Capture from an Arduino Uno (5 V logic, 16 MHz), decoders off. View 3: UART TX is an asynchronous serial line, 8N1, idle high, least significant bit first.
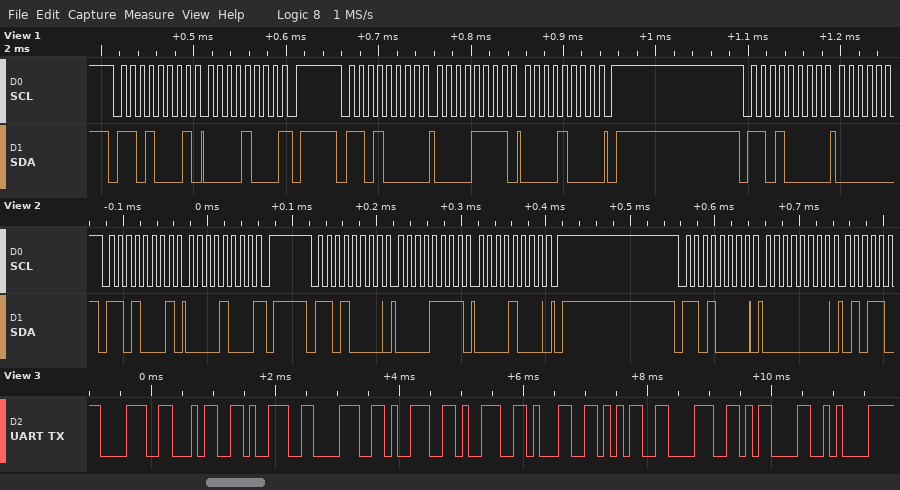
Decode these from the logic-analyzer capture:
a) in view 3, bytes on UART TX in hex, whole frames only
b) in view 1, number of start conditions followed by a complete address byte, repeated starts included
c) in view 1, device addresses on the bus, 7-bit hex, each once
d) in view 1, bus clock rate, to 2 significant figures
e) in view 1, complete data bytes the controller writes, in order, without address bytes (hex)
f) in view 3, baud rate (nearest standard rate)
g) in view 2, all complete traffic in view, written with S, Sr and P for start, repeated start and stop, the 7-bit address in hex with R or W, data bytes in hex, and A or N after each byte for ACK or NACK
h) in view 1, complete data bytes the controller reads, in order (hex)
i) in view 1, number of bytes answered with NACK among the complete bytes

38 34 39 38 39 39 31 35 38 0D 0A
3
0x68
100 kHz
0F 08
9600 baud
S 68R A 08 N P S 68W A 0F A 08 A P S 68W A 00 A
08
1
